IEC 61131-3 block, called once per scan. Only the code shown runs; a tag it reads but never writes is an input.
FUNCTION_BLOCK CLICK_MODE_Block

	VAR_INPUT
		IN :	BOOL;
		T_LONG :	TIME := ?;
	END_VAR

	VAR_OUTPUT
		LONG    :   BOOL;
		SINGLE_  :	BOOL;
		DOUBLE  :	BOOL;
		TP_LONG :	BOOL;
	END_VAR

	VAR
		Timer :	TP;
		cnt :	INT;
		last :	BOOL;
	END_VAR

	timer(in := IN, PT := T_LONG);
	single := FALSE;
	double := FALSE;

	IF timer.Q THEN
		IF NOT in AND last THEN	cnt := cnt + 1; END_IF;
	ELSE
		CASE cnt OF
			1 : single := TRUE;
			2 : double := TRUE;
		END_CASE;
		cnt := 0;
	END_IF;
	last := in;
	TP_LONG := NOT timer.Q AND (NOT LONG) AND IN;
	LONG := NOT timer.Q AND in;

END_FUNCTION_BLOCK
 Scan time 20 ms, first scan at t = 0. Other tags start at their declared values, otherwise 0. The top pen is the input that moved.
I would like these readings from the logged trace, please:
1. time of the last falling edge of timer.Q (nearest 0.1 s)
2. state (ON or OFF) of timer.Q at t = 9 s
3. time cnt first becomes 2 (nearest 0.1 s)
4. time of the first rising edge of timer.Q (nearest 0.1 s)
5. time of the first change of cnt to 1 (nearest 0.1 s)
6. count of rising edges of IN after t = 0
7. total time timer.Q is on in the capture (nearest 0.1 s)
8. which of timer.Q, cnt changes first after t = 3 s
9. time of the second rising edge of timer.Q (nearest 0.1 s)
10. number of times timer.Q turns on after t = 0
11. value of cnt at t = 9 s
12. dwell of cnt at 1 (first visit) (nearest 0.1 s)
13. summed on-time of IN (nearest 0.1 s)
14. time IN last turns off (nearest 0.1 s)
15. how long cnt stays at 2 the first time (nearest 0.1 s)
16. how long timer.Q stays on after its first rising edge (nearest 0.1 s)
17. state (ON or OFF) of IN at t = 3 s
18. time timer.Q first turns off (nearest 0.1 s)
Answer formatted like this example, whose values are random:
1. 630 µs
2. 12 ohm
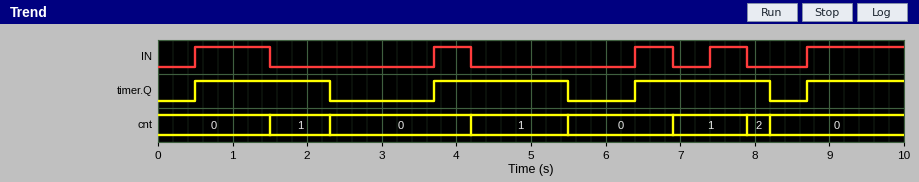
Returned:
1. 8.2 s
2. ON
3. 7.9 s
4. 0.5 s
5. 1.5 s
6. 5
7. 6.7 s
8. timer.Q
9. 3.7 s
10. 4
11. 0
12. 0.8 s
13. 3.8 s
14. 7.9 s
15. 0.3 s
16. 1.8 s
17. OFF
18. 2.3 s
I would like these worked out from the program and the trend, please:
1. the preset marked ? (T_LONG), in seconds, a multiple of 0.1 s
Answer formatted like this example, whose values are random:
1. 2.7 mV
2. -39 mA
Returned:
1. 1.8 s
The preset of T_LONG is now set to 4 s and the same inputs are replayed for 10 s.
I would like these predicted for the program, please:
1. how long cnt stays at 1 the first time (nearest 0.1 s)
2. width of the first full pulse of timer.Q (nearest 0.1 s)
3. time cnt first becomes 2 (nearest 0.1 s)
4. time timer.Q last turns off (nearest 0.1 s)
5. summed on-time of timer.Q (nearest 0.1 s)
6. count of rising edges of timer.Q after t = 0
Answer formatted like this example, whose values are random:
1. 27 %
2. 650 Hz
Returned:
1. 2.7 s
2. 4.0 s
3. 4.2 s
4. 4.5 s
5. 7.6 s
6. 2
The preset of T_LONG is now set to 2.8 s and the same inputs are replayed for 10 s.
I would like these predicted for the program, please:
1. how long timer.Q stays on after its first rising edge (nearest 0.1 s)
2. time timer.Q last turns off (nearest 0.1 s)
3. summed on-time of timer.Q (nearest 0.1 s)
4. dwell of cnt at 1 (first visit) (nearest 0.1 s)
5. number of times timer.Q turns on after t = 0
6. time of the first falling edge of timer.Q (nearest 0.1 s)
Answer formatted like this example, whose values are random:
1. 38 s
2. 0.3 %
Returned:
1. 2.8 s
2. 6.5 s
3. 8.2 s
4. 1.8 s
5. 3
6. 3.3 s
